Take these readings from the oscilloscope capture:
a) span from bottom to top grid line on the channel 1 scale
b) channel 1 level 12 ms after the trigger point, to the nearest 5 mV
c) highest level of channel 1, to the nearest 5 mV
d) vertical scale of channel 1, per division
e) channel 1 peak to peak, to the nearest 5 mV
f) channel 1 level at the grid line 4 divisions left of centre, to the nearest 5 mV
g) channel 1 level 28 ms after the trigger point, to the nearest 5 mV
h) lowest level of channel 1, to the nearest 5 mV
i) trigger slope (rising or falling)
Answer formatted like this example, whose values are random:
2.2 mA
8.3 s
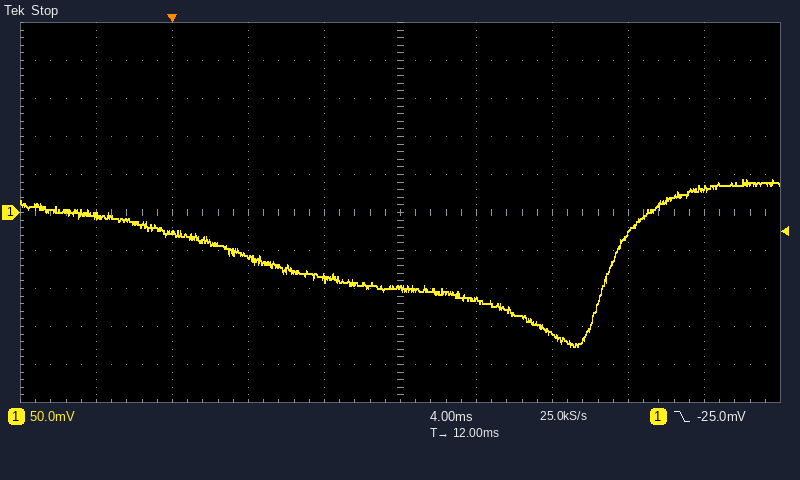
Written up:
500 mV
-100 mV
45 mV
50 mV
220 mV
-5 mV
30 mV
-175 mV
falling
